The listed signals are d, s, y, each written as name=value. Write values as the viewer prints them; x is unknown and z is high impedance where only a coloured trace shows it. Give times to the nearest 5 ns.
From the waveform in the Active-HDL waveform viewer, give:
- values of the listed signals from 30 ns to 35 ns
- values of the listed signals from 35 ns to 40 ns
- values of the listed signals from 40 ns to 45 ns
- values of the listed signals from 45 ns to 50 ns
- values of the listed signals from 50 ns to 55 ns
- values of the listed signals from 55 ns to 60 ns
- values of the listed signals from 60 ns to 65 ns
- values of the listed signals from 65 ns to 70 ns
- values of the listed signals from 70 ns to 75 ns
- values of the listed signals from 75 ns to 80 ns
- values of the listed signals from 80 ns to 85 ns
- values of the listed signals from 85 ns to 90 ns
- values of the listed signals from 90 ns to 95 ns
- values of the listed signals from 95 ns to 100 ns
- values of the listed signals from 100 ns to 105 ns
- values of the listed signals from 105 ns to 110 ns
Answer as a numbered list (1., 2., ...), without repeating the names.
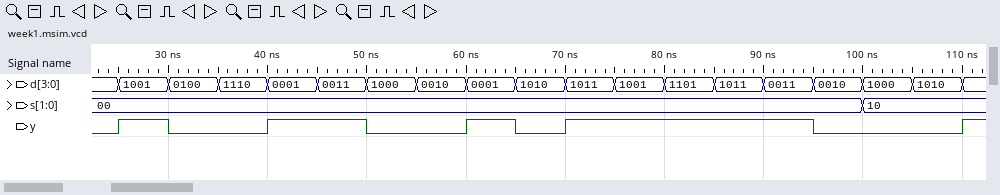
1. d=0100, s=00, y=0
2. d=1110, s=00, y=0
3. d=0001, s=00, y=1
4. d=0011, s=00, y=1
5. d=1000, s=00, y=0
6. d=0010, s=00, y=0
7. d=0001, s=00, y=1
8. d=1010, s=00, y=0
9. d=1011, s=00, y=1
10. d=1001, s=00, y=1
11. d=1101, s=00, y=1
12. d=1011, s=00, y=1
13. d=0011, s=00, y=1
14. d=0010, s=00, y=0
15. d=1000, s=10, y=0
16. d=1010, s=10, y=0
